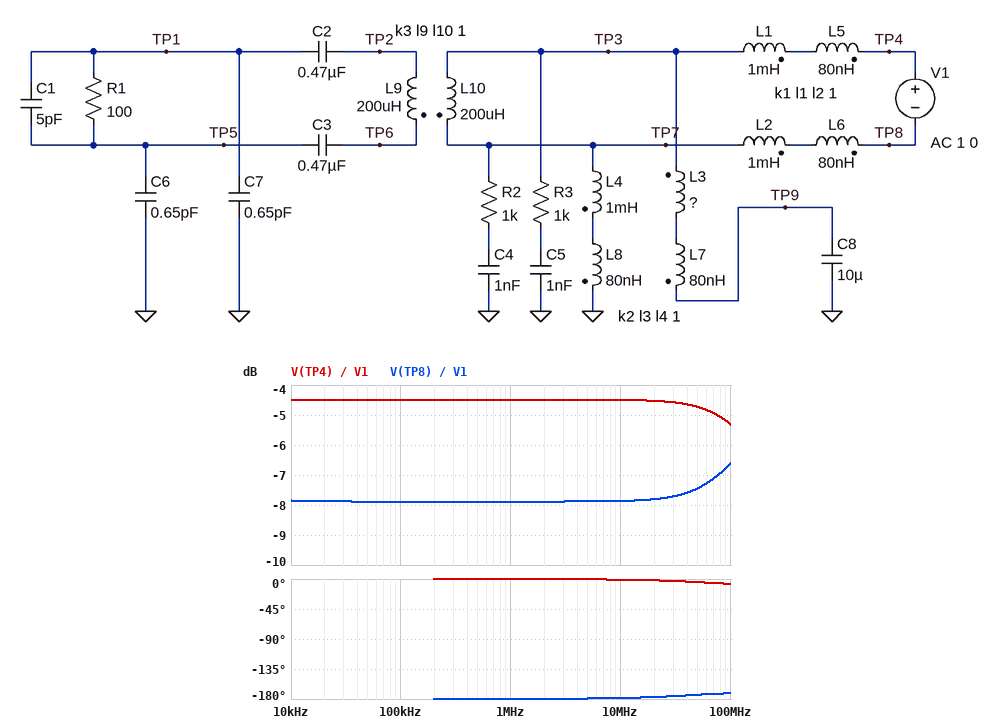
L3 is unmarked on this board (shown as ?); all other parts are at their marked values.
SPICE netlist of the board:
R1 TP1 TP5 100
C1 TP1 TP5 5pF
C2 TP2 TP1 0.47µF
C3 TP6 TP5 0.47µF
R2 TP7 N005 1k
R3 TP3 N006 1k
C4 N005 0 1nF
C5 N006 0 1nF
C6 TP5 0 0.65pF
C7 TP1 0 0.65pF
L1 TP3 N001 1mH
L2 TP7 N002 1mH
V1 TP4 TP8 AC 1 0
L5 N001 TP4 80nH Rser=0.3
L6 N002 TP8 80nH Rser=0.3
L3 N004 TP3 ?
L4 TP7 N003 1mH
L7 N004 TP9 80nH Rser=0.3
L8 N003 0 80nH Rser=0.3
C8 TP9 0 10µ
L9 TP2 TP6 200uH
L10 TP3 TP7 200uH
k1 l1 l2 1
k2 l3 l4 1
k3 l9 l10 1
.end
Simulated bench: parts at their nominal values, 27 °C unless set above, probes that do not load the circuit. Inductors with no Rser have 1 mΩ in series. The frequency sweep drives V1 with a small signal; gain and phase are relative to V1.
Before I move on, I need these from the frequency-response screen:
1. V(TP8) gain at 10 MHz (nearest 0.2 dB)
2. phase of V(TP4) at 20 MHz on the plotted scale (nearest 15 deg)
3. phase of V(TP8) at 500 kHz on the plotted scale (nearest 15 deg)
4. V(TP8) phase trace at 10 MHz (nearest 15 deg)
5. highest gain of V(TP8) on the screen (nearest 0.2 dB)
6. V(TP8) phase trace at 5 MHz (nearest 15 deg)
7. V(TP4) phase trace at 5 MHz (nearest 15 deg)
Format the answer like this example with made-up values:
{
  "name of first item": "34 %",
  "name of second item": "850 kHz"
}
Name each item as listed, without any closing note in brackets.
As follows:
{
  "V(TP8) gain at 10 MHz": "-7.8 dB",
  "phase of V(TP4) at 20 MHz on the plotted scale": "0 deg",
  "phase of V(TP8) at 500 kHz on the plotted scale": "-180 deg",
  "V(TP8) phase trace at 10 MHz": "-180 deg",
  "highest gain of V(TP8) on the screen": "-6.6 dB",
  "V(TP8) phase trace at 5 MHz": "-180 deg",
  "V(TP4) phase trace at 5 MHz": "0 deg"
}
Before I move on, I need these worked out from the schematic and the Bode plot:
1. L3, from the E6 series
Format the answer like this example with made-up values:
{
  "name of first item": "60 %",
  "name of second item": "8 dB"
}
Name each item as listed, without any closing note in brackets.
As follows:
{
  "L3, from the E6 series": "2.2 mH"
}
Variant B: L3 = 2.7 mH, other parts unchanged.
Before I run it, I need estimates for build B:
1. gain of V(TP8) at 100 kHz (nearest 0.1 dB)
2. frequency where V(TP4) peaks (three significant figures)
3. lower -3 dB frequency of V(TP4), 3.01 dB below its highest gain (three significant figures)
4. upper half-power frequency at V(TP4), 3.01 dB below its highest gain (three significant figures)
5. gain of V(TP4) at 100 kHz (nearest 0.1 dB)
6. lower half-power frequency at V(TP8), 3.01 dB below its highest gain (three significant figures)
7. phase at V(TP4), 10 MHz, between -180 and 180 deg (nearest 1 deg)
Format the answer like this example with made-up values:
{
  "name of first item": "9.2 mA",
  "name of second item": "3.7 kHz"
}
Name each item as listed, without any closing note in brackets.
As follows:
{
  "gain of V(TP8) at 100 kHz": "-8.4 dB",
  "frequency where V(TP4) peaks": "598 Hz",
  "lower -3 dB frequency of V(TP4), 3.01 dB below its highest gain": "586 Hz",
  "upper half-power frequency at V(TP4), 3.01 dB below its highest gain": "608 Hz",
  "gain of V(TP4) at 100 kHz": "-4.1 dB",
  "lower half-power frequency at V(TP8), 3.01 dB below its highest gain": "588 Hz",
  "phase at V(TP4), 10 MHz, between -180 and 180 deg": "-1 deg"
}
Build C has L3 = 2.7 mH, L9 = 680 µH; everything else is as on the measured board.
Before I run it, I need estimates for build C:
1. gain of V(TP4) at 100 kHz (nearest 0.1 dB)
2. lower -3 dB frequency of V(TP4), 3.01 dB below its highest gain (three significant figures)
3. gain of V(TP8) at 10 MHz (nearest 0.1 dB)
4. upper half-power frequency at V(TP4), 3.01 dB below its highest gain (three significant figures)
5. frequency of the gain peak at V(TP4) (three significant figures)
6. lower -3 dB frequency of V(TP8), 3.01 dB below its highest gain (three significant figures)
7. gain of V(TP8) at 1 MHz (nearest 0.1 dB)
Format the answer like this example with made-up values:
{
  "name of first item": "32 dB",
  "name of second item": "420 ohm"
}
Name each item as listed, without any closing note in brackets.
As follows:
{
  "gain of V(TP4) at 100 kHz": "-4.2 dB",
  "lower -3 dB frequency of V(TP4), 3.01 dB below its highest gain": "586 Hz",
  "gain of V(TP8) at 10 MHz": "-8.1 dB",
  "upper half-power frequency at V(TP4), 3.01 dB below its highest gain": "608 Hz",
  "frequency of the gain peak at V(TP4)": "598 Hz",
  "lower -3 dB frequency of V(TP8), 3.01 dB below its highest gain": "588 Hz",
  "gain of V(TP8) at 1 MHz": "-8.4 dB"
}
